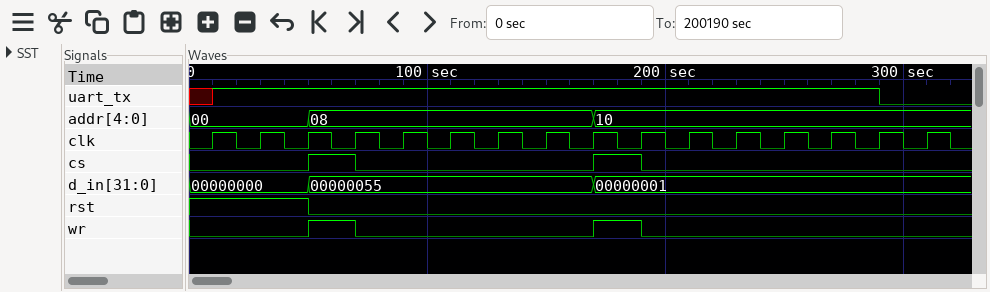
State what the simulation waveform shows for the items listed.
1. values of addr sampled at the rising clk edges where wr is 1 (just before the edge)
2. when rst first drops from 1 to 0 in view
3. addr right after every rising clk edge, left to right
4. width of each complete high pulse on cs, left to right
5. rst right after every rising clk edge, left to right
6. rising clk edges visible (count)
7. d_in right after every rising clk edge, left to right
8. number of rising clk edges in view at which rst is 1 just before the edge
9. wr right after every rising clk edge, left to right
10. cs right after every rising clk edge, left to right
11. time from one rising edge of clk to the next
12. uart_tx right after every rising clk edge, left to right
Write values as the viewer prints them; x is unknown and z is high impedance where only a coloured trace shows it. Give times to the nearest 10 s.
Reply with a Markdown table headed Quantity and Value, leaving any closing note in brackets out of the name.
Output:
| Quantity | Value |
|---|---|
| values of addr sampled at the rising clk edges where wr is 1 | 08, 10 |
| when rst first drops from 1 to 0 in view | 50 s |
| addr right after every rising clk edge, left to right | 00, 00, 08, 08, 08, 08, 08, 08, 10, 10, 10, 10, 10, 10, 10, 10 |
| width of each complete high pulse on cs, left to right | 20 s, 20 s |
| rst right after every rising clk edge, left to right | 1 1 0 0 0 0 0 0 0 0 0 0 0 0 0 0 |
| rising clk edges visible | 16 |
| d_in right after every rising clk edge, left to right | 00000000, 00000000, 00000055, 00000055, 00000055, 00000055, 00000055, 00000055, 00000001, 00000001, 00000001, 00000001, 00000001, 00000001, 00000001, 00000001 |
| number of rising clk edges in view at which rst is 1 just before the edge | 3 |
| wr right after every rising clk edge, left to right | 0 0 1 0 0 0 0 0 1 0 0 0 0 0 0 0 |
| cs right after every rising clk edge, left to right | 0 0 1 0 0 0 0 0 1 0 0 0 0 0 0 0 |
| time from one rising edge of clk to the next | 20 s |
| uart_tx right after every rising clk edge, left to right | 1 1 1 1 1 1 1 1 1 1 1 1 1 1 0 0 |
